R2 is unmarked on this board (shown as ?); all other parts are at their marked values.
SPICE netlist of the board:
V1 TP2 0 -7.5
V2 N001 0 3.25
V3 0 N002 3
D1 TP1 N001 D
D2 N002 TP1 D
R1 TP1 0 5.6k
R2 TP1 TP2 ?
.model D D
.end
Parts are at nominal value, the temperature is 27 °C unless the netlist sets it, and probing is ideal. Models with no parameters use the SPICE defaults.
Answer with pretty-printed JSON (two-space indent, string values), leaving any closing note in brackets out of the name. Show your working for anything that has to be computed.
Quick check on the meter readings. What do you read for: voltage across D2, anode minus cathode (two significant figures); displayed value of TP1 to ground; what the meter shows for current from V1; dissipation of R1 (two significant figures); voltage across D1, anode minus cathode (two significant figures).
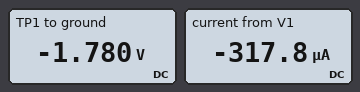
{
  "voltage across D2, anode minus cathode": "-3 V - (-1.78 V) = -1.2 V",
  "displayed value of TP1 to ground": "-1.780 V",
  "what the meter shows for current from V1": "-317.8 µA",
  "dissipation of R1": "(0 V - (-1.78 V))^2 / 5.6 kΩ = 570 µW",
  "voltage across D1, anode minus cathode": "-1.78 V - 3.25 V = -5.0 V"
}
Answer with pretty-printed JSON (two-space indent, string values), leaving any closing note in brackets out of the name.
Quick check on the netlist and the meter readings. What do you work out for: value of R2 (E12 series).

{
  "value of R2": "18 kΩ"
}
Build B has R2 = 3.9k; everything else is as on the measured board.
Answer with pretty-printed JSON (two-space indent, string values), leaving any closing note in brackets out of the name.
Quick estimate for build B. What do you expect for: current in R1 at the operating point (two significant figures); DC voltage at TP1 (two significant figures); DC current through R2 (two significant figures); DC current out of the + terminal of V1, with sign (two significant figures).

{
  "current in R1 at the operating point": "650 µA",
  "DC voltage at TP1": "-3.6 V",
  "DC current through R2": "990 µA",
  "DC current out of the + terminal of V1, with sign": "-990 µA"
}
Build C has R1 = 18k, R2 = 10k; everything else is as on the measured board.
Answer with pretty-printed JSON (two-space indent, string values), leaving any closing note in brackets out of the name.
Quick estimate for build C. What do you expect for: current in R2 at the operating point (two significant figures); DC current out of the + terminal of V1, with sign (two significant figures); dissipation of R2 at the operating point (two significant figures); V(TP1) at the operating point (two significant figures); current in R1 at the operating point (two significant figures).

{
  "current in R2 at the operating point": "390 µA",
  "DC current out of the + terminal of V1, with sign": "-390 µA",
  "dissipation of R2 at the operating point": "1.5 mW",
  "V(TP1) at the operating point": "-3.6 V",
  "current in R1 at the operating point": "200 µA"
}
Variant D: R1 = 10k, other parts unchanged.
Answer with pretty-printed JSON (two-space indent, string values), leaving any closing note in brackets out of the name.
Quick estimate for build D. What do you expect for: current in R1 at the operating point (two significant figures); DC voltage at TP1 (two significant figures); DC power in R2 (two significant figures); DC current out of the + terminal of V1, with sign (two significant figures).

{
  "current in R1 at the operating point": "270 µA",
  "DC voltage at TP1": "-2.7 V",
  "DC power in R2": "1.3 mW",
  "DC current out of the + terminal of V1, with sign": "-270 µA"
}
